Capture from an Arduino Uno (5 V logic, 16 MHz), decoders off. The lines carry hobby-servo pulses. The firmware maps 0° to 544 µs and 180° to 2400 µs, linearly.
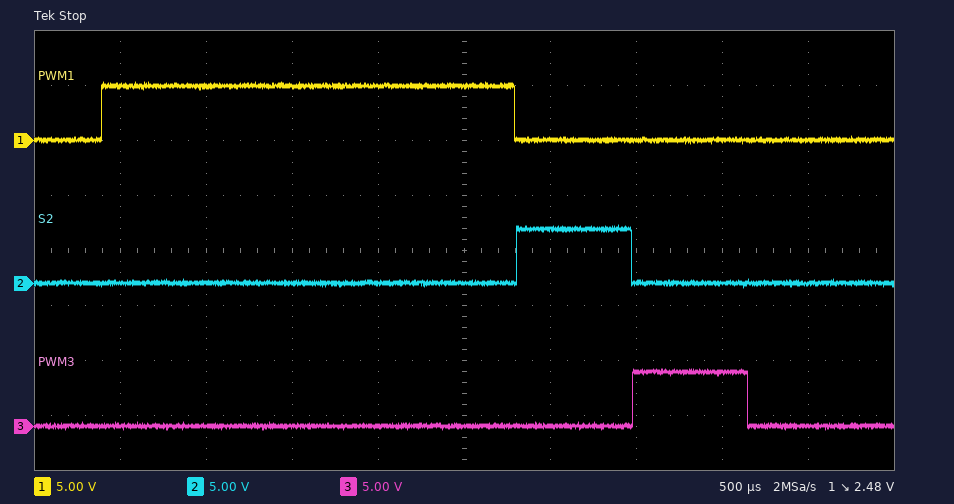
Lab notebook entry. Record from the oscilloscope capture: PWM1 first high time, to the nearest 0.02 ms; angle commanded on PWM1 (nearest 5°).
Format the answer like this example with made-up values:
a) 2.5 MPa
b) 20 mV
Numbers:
a) 2.40 ms
b) 180°
